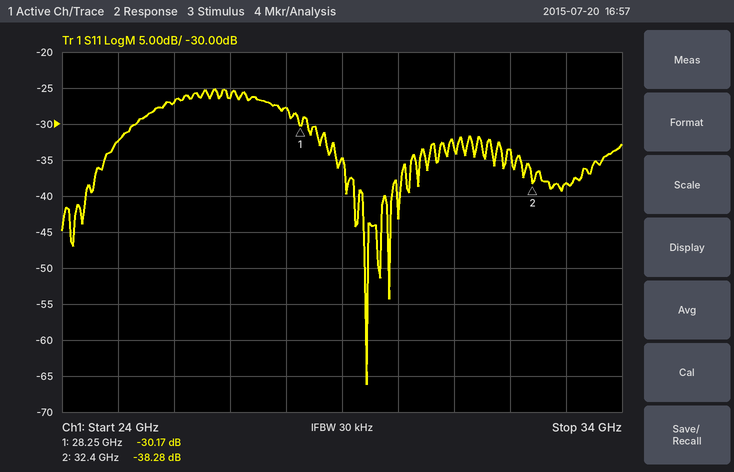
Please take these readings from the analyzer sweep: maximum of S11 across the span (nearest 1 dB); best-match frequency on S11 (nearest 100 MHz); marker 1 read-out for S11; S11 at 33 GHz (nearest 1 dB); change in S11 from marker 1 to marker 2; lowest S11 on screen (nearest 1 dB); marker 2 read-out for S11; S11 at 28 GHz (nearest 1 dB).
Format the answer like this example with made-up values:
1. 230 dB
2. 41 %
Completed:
1. -25 dB
2. 29.4 GHz
3. -30.17 dB
4. -38 dB
5. -8.11 dB
6. -66 dB
7. -38.28 dB
8. -28 dB
